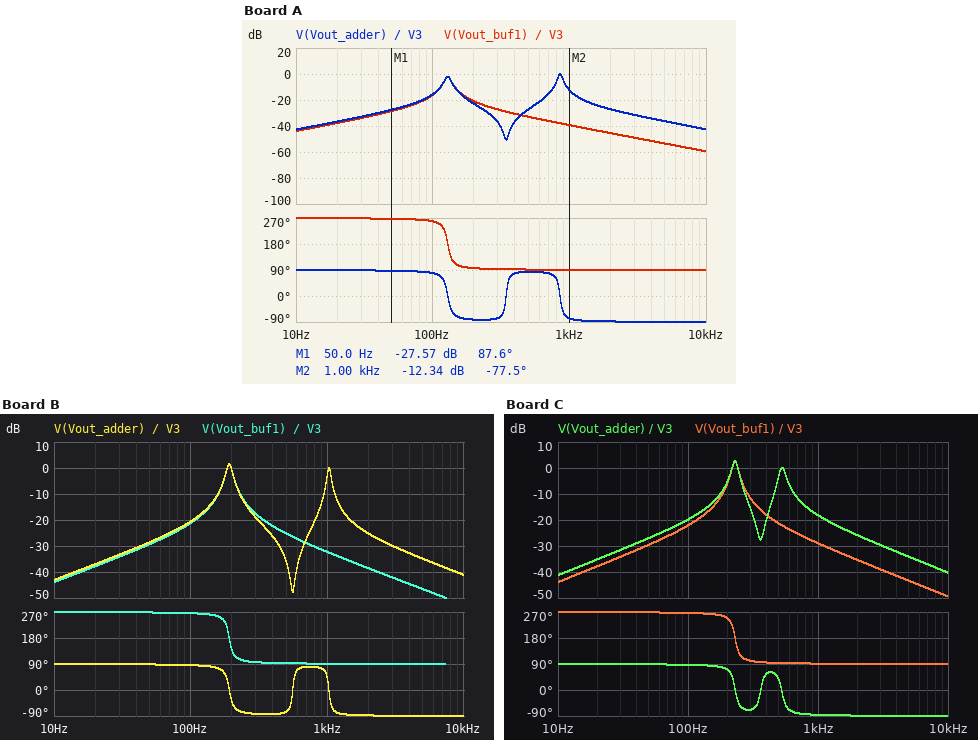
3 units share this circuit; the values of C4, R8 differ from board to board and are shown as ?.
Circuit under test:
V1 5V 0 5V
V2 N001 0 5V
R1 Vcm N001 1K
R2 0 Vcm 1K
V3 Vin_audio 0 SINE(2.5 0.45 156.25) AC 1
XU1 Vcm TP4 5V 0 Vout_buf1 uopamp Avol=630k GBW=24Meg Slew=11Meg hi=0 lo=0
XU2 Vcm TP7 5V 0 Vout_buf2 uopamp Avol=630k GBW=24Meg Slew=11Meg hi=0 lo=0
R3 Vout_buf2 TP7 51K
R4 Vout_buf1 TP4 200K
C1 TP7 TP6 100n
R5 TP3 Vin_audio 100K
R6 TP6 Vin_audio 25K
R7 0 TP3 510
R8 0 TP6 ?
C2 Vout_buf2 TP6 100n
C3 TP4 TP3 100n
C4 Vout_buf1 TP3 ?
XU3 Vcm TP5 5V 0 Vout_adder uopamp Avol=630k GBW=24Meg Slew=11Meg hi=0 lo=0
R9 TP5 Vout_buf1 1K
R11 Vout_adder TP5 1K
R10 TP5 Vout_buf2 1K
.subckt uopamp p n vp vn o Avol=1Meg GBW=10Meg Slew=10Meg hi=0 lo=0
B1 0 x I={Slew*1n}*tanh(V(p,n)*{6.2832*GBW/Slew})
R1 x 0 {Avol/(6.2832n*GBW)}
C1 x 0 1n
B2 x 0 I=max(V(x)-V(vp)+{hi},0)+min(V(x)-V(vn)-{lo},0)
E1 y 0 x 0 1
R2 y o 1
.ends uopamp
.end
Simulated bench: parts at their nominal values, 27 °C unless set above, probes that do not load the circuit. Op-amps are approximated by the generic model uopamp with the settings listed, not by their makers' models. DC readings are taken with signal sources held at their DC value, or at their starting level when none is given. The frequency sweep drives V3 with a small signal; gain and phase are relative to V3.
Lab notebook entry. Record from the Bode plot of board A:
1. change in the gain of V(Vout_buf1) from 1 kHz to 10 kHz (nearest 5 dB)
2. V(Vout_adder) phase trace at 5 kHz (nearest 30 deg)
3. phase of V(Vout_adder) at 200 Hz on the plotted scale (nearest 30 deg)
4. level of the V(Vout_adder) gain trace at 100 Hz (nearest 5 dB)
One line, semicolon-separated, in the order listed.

-20 dB; -90 deg; -90 deg; -15 dB
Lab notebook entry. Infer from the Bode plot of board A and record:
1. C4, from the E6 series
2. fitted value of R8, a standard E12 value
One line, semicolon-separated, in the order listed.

150 nF; 68 Ω
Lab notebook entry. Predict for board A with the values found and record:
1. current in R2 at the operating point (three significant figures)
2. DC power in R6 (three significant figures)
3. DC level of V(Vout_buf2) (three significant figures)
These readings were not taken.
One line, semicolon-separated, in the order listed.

2.50 mA; 249 µW; 2.50 V
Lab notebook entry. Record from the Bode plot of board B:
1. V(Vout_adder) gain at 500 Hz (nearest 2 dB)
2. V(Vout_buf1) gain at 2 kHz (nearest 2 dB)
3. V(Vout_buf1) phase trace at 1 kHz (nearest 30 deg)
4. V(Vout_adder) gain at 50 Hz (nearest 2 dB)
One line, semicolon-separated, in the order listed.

-36 dB; -38 dB; 90 deg; -28 dB
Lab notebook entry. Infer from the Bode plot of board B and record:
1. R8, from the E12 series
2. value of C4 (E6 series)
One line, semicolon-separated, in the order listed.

47 Ω; 68 nF
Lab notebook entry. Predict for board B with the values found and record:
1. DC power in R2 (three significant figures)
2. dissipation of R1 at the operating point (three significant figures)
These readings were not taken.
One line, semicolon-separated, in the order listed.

6.25 mW; 6.25 mW
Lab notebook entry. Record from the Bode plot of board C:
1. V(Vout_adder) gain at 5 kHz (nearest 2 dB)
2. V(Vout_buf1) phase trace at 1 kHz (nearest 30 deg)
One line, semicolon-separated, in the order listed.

-34 dB; 90 deg
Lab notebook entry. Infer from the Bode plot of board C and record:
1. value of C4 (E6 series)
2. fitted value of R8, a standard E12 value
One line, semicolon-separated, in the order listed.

47 nF; 180 Ω
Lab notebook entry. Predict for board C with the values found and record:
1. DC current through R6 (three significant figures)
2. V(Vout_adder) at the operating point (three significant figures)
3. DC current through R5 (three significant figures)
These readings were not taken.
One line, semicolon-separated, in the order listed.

99.3 µA; 2.50 V; 24.9 µA
